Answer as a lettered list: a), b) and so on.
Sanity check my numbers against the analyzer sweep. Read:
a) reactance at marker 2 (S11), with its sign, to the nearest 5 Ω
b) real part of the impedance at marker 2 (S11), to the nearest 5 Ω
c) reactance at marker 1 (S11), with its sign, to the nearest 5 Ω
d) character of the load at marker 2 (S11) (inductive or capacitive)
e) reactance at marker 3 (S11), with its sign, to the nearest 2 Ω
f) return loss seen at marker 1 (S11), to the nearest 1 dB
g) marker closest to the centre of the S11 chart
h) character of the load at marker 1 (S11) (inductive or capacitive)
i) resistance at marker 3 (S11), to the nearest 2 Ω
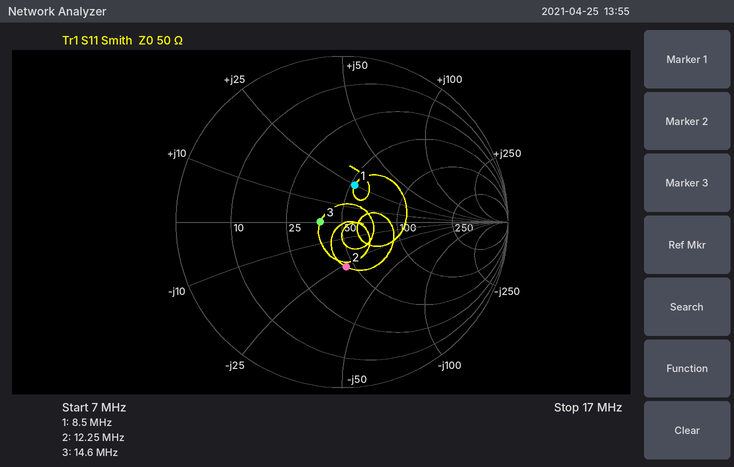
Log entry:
a) -25 Ω
b) 45 Ω
c) +25 Ω
d) capacitive
e) 0 Ω
f) 13 dB
g) marker 3
h) inductive
i) 38 Ω
